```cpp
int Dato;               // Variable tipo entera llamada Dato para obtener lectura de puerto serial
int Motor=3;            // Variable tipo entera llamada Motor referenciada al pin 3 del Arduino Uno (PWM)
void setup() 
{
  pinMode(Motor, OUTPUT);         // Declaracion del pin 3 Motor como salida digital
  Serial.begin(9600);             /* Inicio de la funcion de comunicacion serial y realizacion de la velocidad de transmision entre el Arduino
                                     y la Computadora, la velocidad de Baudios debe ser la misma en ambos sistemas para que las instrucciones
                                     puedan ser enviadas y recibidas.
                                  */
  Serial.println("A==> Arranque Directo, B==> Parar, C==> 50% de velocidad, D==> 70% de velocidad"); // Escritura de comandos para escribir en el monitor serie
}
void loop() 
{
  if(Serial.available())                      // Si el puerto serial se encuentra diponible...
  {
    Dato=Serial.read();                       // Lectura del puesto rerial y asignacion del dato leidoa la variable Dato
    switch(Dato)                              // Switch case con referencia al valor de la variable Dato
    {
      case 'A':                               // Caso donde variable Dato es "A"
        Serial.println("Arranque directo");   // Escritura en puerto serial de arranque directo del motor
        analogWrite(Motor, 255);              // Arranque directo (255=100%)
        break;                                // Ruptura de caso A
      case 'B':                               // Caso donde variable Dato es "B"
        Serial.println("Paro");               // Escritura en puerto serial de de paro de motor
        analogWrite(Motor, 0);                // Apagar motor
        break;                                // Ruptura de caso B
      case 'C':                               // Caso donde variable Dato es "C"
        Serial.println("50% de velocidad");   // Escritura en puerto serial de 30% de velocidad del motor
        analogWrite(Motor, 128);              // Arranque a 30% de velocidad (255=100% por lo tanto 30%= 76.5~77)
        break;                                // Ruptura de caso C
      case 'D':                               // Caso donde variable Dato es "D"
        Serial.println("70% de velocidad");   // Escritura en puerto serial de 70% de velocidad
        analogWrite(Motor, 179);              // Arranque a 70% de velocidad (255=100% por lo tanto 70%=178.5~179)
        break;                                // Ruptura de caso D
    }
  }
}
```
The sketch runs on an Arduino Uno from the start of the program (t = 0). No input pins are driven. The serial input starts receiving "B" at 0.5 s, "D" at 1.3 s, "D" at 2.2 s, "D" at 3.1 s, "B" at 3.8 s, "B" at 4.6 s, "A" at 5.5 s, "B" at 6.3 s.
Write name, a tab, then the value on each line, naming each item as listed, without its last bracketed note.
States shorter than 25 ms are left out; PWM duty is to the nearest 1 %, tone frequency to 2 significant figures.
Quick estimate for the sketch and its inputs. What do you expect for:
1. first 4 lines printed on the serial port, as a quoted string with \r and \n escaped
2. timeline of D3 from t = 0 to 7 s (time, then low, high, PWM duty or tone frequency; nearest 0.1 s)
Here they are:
first 4 lines printed on the serial port, as a quoted string with \r and \n escaped	"A==> Arranque Directo, B==> Parar, C==> 50% de velocidad, D==> 70% de velocidad\r\nParo\r\n70% de velocidad\r\n70% de velocidad\r\n"
timeline of D3 from t = 0 to 7 s	0 s low; 1.3 s PWM 70 %; 3.8 s low; 5.5 s high; 6.3 s low
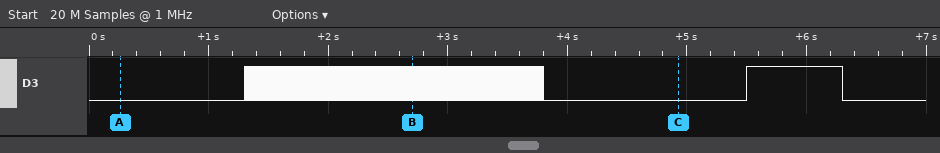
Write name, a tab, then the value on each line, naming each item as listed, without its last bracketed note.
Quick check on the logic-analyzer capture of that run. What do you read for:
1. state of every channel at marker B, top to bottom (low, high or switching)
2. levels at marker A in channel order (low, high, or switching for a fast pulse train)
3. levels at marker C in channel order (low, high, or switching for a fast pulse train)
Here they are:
state of every channel at marker B, top to bottom	D3 switching
levels at marker A in channel order	D3 low
levels at marker C in channel order	D3 low
